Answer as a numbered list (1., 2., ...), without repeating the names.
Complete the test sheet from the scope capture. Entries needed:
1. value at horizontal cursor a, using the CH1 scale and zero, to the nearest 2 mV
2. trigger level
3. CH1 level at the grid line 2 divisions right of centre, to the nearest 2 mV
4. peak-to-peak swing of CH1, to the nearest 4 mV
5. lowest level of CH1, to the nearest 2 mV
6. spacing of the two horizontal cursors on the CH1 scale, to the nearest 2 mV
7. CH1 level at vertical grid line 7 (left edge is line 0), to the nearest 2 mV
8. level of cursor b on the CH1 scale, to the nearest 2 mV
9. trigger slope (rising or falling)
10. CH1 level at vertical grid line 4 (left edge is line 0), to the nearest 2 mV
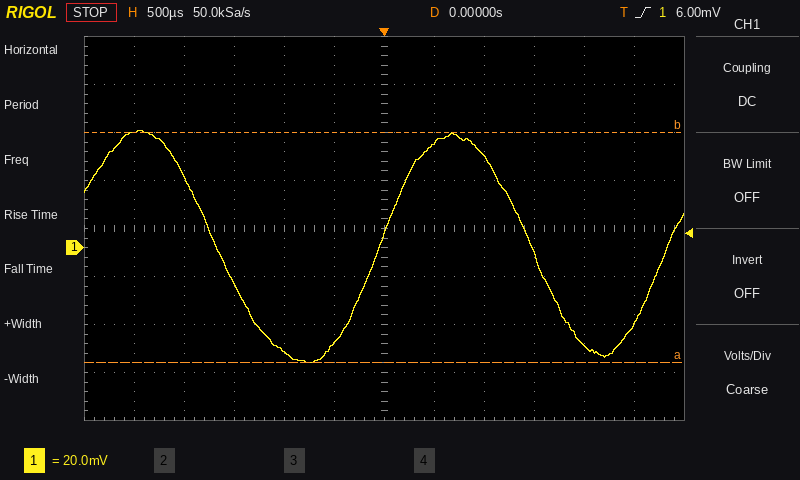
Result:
1. -48 mV
2. 6.00 mV
3. 38 mV
4. 96 mV
5. -48 mV
6. 96 mV
7. 44 mV
8. 48 mV
9. rising
10. -44 mV
